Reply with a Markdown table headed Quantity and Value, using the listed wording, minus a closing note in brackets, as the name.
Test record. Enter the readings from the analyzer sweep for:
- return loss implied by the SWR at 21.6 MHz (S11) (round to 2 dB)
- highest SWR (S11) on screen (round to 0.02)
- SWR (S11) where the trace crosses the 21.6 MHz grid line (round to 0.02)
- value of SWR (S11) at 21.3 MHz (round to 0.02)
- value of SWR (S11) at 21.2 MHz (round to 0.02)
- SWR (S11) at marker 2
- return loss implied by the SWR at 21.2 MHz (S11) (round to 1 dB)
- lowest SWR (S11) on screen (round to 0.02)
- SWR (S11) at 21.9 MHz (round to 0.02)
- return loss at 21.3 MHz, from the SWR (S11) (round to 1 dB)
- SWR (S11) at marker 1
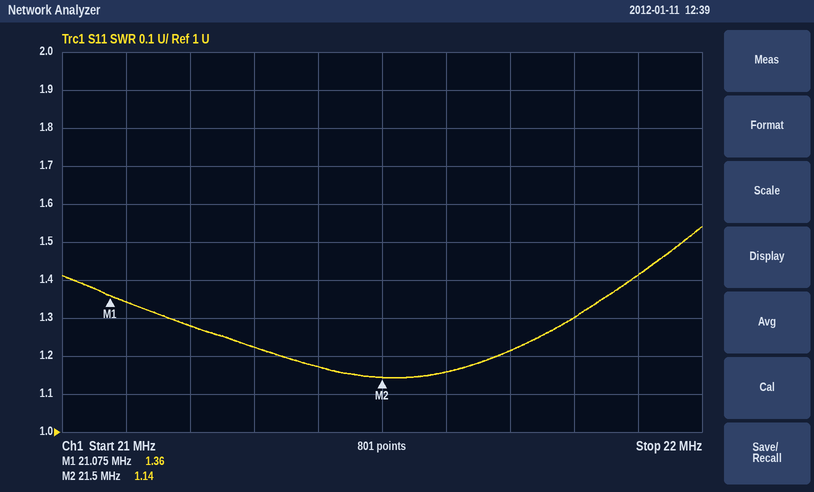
| Quantity | Value |
|---|---|
| return loss implied by the SWR at 21.6 MHz (S11) | 22 dB |
| highest SWR (S11) on screen | 1.54 |
| SWR (S11) where the trace crosses the 21.6 MHz grid line | 1.16 |
| value of SWR (S11) at 21.3 MHz | 1.22 |
| value of SWR (S11) at 21.2 MHz | 1.28 |
| SWR (S11) at marker 2 | 1.14 |
| return loss implied by the SWR at 21.2 MHz (S11) | 18 dB |
| lowest SWR (S11) on screen | 1.14 |
| SWR (S11) at 21.9 MHz | 1.42 |
| return loss at 21.3 MHz, from the SWR (S11) | 20 dB |
| SWR (S11) at marker 1 | 1.36 |
